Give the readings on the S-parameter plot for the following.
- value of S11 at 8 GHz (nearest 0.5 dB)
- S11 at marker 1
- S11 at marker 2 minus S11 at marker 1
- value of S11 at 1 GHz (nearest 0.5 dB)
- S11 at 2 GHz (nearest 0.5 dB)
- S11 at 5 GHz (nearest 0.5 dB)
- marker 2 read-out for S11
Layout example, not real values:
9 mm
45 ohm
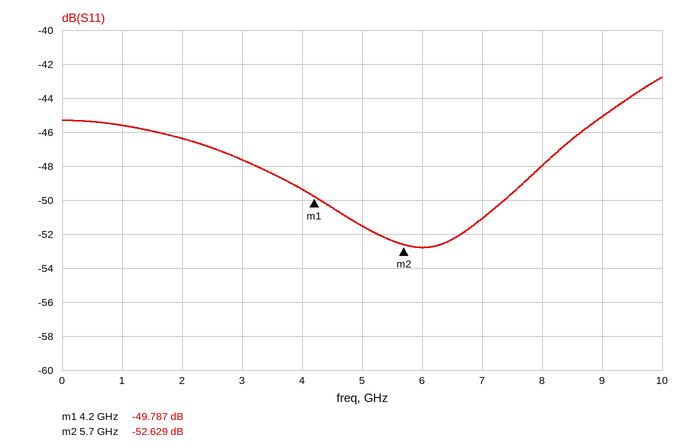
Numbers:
-48.0 dB
-49.787 dB
-2.842 dB
-45.5 dB
-46.5 dB
-51.5 dB
-52.629 dB
